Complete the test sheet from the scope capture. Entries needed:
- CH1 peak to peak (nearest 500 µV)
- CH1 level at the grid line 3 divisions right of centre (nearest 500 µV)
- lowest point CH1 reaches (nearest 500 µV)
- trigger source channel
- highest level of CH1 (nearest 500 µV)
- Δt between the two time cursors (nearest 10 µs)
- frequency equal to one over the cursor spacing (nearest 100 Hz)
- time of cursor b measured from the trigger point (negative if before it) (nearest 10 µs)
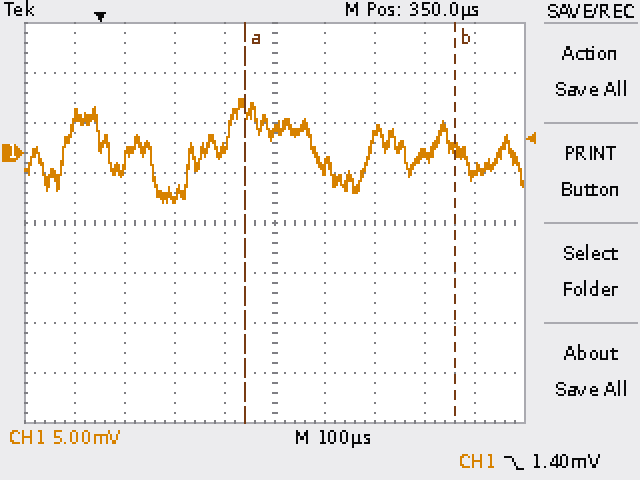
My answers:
10.5 mV
0.0 mV
-5.0 mV
CH1
5.5 mV
420 µs
2.4 kHz
+710 µs
